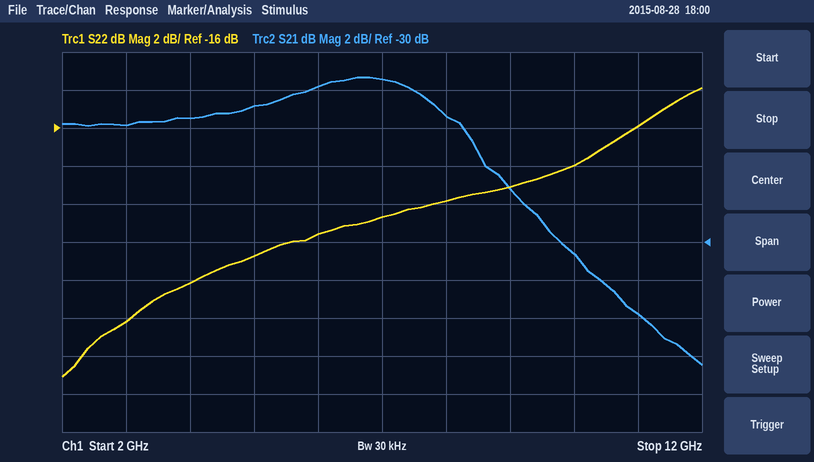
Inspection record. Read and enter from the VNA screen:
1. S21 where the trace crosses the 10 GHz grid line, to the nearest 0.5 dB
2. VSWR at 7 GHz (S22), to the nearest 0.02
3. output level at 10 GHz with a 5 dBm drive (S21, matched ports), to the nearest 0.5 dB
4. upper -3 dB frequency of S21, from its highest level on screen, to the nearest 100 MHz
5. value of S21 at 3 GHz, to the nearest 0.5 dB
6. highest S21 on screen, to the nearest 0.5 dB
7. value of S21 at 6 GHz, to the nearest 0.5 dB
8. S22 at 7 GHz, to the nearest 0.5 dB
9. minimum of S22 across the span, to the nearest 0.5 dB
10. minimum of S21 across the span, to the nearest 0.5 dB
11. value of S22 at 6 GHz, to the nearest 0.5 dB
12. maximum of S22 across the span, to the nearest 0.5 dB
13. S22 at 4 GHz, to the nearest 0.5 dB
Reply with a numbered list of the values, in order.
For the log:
1. -30.5 dB
2. 1.20
3. -25.5 dBm
4. 8.3 GHz
5. -24.0 dB
6. -21.5 dB
7. -22.0 dB
8. -20.5 dB
9. -29.0 dB
10. -36.5 dB
11. -21.5 dB
12. -14.0 dB
13. -24.0 dB
